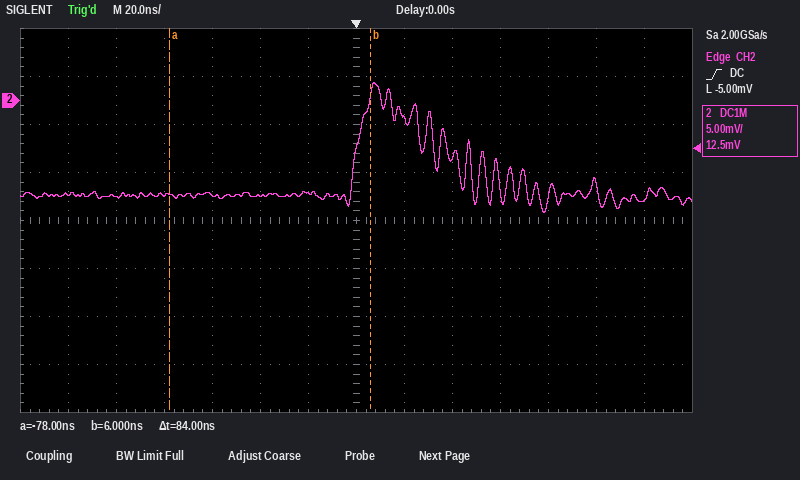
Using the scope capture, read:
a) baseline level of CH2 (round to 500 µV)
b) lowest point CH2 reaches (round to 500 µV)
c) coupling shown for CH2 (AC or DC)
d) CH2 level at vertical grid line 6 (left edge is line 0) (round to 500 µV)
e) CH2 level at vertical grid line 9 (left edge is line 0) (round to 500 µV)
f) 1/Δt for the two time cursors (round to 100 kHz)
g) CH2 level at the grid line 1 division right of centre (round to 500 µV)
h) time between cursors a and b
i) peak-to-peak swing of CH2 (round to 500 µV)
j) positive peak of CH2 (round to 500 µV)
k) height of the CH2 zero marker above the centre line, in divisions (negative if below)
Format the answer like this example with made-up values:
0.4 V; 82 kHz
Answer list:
-10.0 mV; -11.5 mV; DC; -9.5 mV; -6.0 mV; 11.9 MHz; -2.0 mV; 84 ns; 13.5 mV; 2.0 mV; +2.5 div
